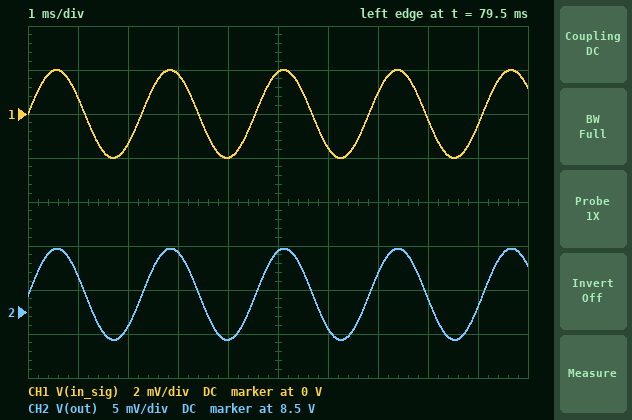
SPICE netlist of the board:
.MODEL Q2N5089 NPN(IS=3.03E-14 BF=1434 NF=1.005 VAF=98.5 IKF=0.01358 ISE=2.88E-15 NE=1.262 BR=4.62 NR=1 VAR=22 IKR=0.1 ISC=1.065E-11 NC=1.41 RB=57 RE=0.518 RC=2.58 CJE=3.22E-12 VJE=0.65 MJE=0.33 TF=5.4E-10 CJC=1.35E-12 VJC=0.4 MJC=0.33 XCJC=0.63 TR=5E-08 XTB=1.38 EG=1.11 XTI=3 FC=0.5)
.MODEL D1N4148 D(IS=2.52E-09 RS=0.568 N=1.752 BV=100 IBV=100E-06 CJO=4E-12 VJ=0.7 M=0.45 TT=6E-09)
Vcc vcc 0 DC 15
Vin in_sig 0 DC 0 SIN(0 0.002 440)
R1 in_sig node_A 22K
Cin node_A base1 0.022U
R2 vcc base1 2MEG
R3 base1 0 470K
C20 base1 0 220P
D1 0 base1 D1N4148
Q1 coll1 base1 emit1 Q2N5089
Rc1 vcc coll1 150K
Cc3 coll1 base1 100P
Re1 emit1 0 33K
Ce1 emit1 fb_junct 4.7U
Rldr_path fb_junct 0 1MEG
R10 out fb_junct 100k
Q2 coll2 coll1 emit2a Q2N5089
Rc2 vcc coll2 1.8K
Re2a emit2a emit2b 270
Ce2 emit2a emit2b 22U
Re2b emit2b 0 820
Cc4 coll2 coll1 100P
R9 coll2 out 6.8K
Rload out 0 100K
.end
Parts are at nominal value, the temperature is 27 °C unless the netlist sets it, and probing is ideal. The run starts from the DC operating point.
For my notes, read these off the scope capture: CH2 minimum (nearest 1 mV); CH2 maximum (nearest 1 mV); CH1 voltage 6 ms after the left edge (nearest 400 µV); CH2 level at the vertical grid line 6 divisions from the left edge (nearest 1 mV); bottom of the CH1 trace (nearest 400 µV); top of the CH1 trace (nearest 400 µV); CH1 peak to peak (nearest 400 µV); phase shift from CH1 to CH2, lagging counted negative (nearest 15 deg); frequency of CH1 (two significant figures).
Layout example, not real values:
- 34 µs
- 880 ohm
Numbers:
- 8.497 V
- 8.507 V
- -1.6 mV
- 8.498 V
- -2.0 mV
- 2.0 mV
- 4.0 mV
- 0 deg
- 440 Hz
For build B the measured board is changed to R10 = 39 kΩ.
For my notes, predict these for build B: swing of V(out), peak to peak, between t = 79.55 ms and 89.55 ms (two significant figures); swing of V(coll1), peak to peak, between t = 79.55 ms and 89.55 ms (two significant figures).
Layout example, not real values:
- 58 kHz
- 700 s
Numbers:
- 6.9 mV
- 3.8 mV
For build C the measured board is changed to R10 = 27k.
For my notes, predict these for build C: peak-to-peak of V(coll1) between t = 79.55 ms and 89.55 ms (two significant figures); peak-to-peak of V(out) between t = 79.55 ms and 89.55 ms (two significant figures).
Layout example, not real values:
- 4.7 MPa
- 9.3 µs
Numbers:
- 3.4 mV
- 6.0 mV
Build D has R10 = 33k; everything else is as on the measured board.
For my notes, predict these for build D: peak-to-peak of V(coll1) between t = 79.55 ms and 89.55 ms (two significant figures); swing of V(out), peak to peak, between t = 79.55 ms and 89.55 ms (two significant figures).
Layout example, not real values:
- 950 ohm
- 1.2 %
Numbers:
- 3.6 mV
- 6.5 mV
